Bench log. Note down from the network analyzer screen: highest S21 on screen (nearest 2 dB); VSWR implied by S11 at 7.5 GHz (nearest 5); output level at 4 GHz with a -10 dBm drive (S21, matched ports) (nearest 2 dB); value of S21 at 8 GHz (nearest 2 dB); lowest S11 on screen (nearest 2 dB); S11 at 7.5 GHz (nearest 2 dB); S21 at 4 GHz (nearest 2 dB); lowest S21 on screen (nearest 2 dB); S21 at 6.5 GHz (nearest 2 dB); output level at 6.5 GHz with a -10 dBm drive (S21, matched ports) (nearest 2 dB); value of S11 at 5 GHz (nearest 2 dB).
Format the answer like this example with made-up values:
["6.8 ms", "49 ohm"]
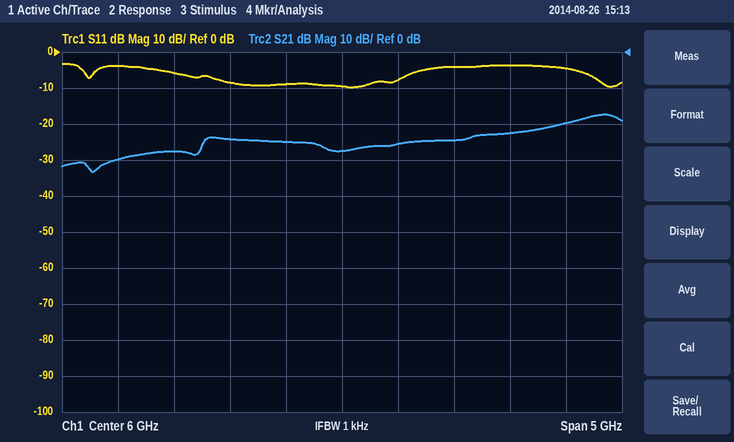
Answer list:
["-18 dB", "5", "-40 dBm", "-20 dB", "-10 dB", "-4 dB", "-30 dB", "-34 dB", "-26 dB", "-36 dBm", "-8 dB"]
